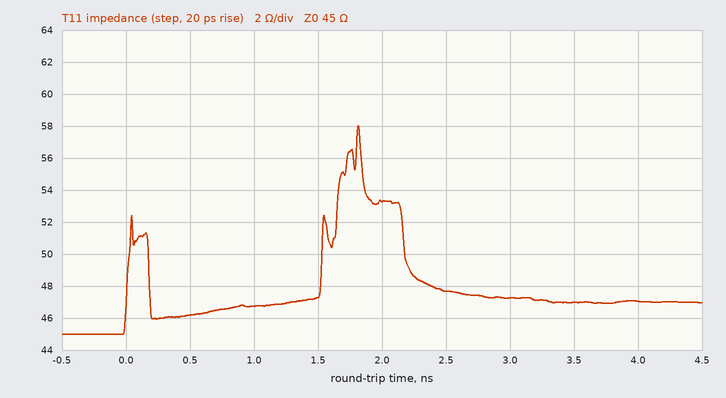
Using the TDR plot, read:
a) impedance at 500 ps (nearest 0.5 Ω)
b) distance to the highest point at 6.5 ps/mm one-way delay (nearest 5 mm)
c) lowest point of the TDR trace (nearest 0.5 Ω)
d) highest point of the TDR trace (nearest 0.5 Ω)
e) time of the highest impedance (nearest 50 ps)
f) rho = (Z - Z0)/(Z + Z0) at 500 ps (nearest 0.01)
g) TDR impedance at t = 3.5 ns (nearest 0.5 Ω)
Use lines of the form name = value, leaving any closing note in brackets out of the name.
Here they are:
impedance at 500 ps = 46.0 Ω
distance to the highest point at 6.5 ps/mm one-way delay = 140 mm
lowest point of the TDR trace = 45.0 Ω
highest point of the TDR trace = 58.0 Ω
time of the highest impedance = 1.80 ns
rho = (Z - Z0)/(Z + Z0) at 500 ps = +0.01
TDR impedance at t = 3.5 ns = 47.0 Ω
